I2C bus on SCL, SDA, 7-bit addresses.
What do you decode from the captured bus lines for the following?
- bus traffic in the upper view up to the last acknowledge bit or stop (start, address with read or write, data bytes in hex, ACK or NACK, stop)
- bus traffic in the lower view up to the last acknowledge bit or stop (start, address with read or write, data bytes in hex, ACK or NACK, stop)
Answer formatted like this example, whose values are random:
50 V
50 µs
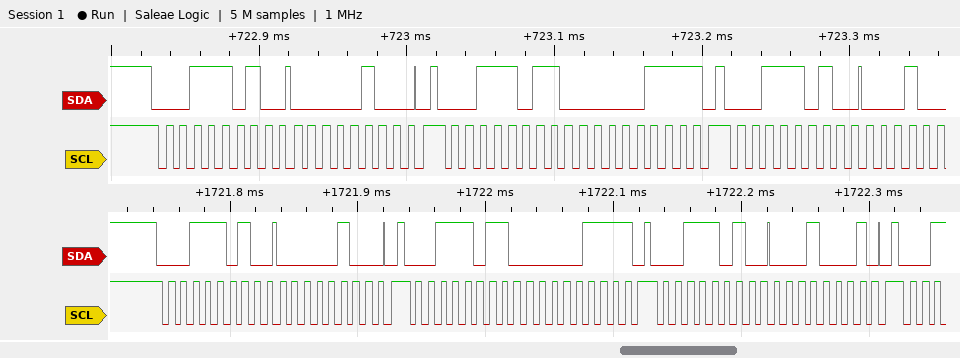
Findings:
start, address 1D write ACK, 04 ACK, stop, start, address 1D read ACK, 07 NACK, stop, start, address 1D write ACK
start, address 1D write ACK, 04 ACK, stop, start, address 1D read ACK, 07 NACK, stop, start, address 1D write ACK, 11 ACK, stop
